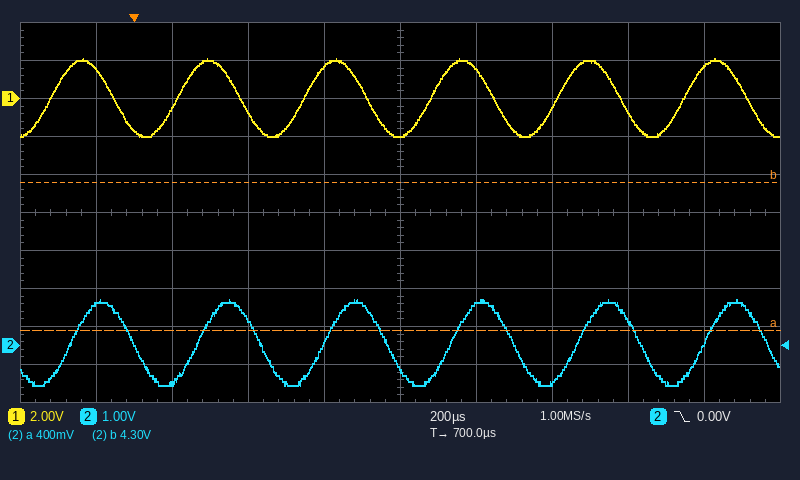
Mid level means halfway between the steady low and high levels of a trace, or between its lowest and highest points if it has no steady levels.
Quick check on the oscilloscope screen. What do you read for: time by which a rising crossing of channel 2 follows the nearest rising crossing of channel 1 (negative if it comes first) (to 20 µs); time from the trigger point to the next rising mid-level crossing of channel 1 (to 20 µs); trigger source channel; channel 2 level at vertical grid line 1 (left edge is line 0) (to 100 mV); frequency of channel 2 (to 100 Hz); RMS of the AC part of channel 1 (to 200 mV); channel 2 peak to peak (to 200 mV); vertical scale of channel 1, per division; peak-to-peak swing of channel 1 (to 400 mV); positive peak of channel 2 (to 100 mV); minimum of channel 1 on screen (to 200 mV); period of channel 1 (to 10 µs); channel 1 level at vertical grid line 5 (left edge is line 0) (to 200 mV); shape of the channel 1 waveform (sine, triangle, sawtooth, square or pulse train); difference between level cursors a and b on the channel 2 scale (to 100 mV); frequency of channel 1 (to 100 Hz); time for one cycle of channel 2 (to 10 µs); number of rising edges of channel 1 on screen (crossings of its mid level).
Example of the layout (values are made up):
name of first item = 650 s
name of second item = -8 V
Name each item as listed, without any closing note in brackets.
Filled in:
time by which a rising crossing of channel 2 follows the nearest rising crossing of channel 1 (negative if it comes first) = +60 µs
time from the trigger point to the next rising mid-level crossing of channel 1 = 120 µs
trigger source channel = channel 2
channel 2 level at vertical grid line 1 (left edge is line 0) = 1.1 V
frequency of channel 2 = 3.0 kHz
RMS of the AC part of channel 1 = 1.4 V
channel 2 peak to peak = 2.2 V
vertical scale of channel 1, per division = 2 V
peak-to-peak swing of channel 1 = 4.0 V
positive peak of channel 2 = 1.2 V
minimum of channel 1 on screen = -2.0 V
period of channel 1 = 330 µs
channel 1 level at vertical grid line 5 (left edge is line 0) = -2.0 V
shape of the channel 1 waveform = sine
difference between level cursors a and b on the channel 2 scale = 3.9 V
frequency of channel 1 = 3.0 kHz
time for one cycle of channel 2 = 330 µs
number of rising edges of channel 1 on screen = 6
